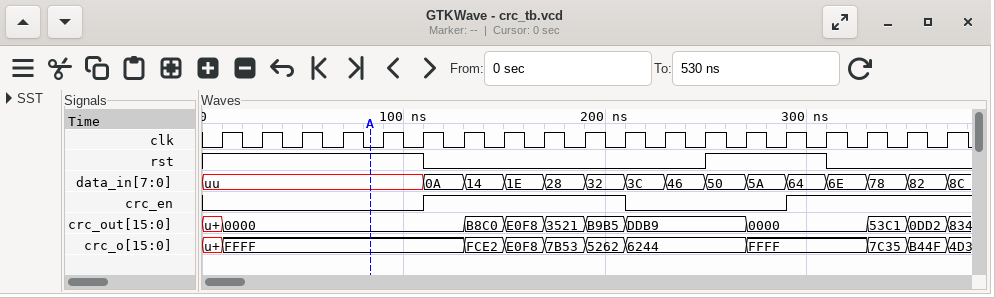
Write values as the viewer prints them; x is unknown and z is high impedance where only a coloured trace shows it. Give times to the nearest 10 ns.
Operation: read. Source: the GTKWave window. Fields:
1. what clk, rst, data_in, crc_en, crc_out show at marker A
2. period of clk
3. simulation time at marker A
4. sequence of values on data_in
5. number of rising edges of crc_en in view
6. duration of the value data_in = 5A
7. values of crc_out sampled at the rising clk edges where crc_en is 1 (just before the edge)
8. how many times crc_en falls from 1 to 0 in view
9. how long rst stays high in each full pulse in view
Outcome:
clk=0, rst=1, data_in=uu, crc_en=0, crc_out=0000
20 ns
80 ns
uu, 0A, 14, 1E, 28, 32, 3C, 46, 50, 5A, 64, 6E, 78, 82, 8C
2
20 ns
0000, B8C0, E0F8, 3521, B9B5, 0000, 0000, 53C1, 0DD2
1
60 ns
